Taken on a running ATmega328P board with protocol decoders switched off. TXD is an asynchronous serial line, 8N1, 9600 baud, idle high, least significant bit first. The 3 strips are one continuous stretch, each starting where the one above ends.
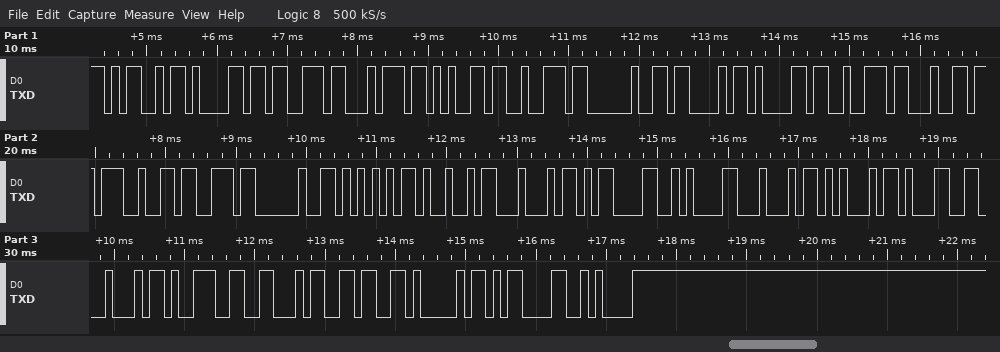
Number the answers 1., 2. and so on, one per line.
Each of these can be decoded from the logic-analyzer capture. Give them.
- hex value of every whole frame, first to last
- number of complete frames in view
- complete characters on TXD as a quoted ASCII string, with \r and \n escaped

1. 0x4D 0x61 0x73 0x74 0x65 0x72 0x20 0x43 0x61 0x72 0x64 0x27 0x73 0x20 0x55 0x49 0x44 0x0D 0x0A 0x44 0x45 0x31 0x44 0x39 0x46 0x36 0x41 0x0D 0x0A
2. 29
3. "Master Card's UID\r\nDE1D9F6A\r\n"
